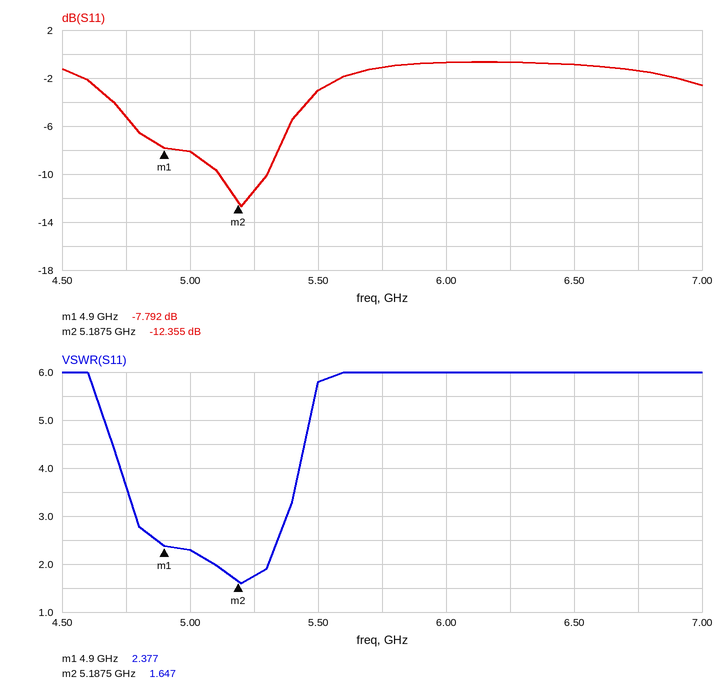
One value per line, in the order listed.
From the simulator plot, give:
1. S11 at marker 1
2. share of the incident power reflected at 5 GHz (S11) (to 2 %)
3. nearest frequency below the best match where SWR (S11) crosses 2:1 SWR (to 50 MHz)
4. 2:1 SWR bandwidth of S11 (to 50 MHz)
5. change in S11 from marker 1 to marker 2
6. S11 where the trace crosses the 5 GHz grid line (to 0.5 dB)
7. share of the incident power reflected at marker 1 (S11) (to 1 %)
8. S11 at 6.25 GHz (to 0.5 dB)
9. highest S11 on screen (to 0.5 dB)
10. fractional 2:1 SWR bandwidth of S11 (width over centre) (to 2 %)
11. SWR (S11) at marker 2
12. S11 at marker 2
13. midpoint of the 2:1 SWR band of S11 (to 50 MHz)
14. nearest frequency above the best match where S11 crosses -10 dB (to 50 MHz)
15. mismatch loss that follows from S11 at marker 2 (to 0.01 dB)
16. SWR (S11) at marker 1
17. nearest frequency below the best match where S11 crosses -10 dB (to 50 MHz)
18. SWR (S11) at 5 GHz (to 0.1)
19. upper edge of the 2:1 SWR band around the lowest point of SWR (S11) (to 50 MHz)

-7.792 dB
16 %
5.10 GHz
200 MHz
-4.563 dB
-8.0 dB
17 %
-0.5 dB
-0.5 dB
4 %
1.647
-12.355 dB
5.20 GHz
5.30 GHz
0.26 dB
2.377
5.10 GHz
2.3
5.30 GHz
